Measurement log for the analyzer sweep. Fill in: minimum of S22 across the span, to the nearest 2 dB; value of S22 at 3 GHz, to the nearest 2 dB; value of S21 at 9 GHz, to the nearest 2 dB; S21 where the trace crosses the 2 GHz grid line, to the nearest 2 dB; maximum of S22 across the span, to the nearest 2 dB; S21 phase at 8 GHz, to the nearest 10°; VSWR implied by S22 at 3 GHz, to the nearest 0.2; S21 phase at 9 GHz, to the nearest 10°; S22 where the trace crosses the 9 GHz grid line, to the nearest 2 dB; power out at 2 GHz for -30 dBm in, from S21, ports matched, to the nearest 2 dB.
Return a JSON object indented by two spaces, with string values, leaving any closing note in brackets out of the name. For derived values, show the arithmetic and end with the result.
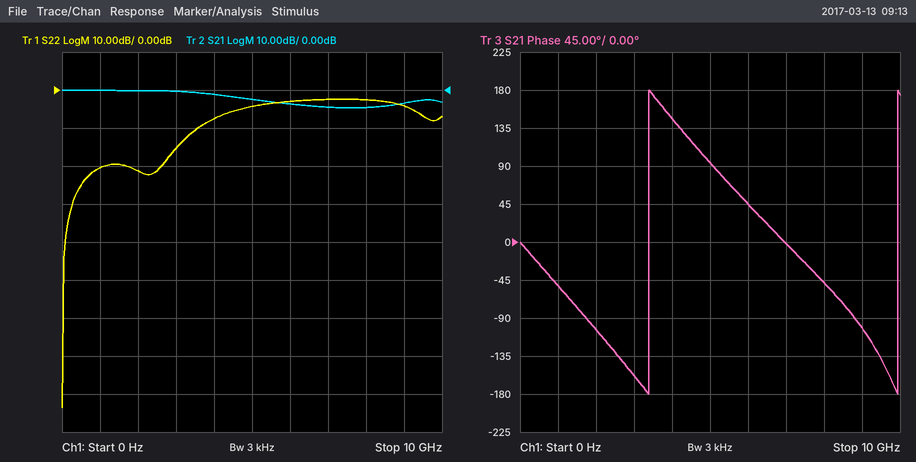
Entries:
{
  "minimum of S22 across the span, to the nearest 2 dB": "-84 dB",
  "value of S22 at 3 GHz, to the nearest 2 dB": "-16 dB",
  "value of S21 at 9 GHz, to the nearest 2 dB": "-4 dB",
  "S21 where the trace crosses the 2 GHz grid line, to the nearest 2 dB": "0 dB",
  "maximum of S22 across the span, to the nearest 2 dB": "-2 dB",
  "S21 phase at 8 GHz, to the nearest 10°": "-50°",
  "VSWR implied by S22 at 3 GHz, to the nearest 0.2": "|Γ| = 10^(-16/20) = 0.1585; VSWR = (1 + 0.1585)/(1 − 0.1585) ≈ 1.4",
  "S21 phase at 9 GHz, to the nearest 10°": "-100°",
  "S22 where the trace crosses the 9 GHz grid line, to the nearest 2 dB": "-4 dB",
  "power out at 2 GHz for -30 dBm in, from S21, ports matched, to the nearest 2 dB": "-30 dBm + (0 dB) = -30 dBm"
}
